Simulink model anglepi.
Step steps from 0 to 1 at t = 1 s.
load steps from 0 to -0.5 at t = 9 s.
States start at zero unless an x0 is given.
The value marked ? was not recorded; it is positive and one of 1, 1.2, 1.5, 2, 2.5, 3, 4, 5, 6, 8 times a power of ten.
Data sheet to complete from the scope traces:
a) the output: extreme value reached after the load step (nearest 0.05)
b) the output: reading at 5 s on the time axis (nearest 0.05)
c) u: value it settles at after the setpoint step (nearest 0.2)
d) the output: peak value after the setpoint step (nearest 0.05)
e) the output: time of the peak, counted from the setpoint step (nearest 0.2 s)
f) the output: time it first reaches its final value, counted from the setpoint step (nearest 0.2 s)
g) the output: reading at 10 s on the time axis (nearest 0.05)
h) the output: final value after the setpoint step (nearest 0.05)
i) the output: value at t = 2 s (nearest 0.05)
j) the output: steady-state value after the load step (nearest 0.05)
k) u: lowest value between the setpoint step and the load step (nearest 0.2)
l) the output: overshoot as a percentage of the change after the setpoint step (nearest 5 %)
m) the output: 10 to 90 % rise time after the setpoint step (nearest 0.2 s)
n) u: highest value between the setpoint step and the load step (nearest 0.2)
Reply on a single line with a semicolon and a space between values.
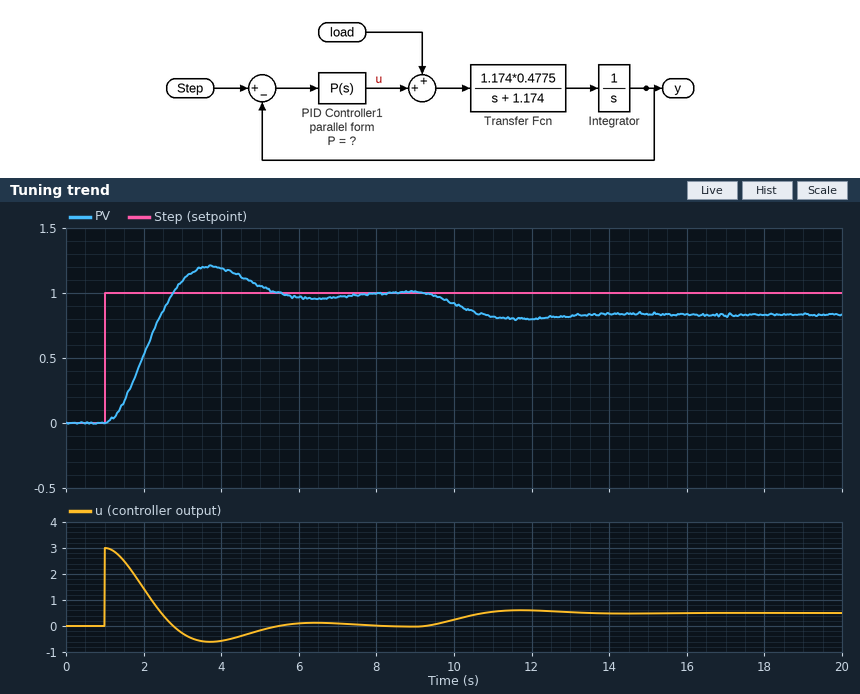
0.80; 1.05; 0.0; 1.20; 2.8 s; 1.8 s; 0.90; 1.00; 0.50; 0.85; -0.6; 20 %; 1.2 s; 3.0
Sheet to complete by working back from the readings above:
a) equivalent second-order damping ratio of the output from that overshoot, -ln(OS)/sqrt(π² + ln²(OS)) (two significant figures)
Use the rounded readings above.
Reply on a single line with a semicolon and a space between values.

0.46
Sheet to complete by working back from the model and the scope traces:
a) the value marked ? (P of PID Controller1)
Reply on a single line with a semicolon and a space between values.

3
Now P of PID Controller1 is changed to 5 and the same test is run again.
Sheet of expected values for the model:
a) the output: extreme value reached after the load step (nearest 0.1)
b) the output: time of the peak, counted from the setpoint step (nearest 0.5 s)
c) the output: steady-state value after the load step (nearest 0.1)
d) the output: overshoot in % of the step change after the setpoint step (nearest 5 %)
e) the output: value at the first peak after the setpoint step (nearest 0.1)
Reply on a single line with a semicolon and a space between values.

0.9; 2.0 s; 0.9; 30 %; 1.3
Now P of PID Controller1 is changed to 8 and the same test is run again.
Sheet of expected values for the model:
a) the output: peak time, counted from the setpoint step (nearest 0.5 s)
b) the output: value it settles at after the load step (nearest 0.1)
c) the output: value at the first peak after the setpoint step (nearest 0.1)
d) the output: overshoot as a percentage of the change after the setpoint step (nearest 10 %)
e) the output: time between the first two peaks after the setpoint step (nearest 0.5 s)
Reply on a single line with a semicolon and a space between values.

1.5 s; 0.9; 1.4; 40 %; 3.0 s
